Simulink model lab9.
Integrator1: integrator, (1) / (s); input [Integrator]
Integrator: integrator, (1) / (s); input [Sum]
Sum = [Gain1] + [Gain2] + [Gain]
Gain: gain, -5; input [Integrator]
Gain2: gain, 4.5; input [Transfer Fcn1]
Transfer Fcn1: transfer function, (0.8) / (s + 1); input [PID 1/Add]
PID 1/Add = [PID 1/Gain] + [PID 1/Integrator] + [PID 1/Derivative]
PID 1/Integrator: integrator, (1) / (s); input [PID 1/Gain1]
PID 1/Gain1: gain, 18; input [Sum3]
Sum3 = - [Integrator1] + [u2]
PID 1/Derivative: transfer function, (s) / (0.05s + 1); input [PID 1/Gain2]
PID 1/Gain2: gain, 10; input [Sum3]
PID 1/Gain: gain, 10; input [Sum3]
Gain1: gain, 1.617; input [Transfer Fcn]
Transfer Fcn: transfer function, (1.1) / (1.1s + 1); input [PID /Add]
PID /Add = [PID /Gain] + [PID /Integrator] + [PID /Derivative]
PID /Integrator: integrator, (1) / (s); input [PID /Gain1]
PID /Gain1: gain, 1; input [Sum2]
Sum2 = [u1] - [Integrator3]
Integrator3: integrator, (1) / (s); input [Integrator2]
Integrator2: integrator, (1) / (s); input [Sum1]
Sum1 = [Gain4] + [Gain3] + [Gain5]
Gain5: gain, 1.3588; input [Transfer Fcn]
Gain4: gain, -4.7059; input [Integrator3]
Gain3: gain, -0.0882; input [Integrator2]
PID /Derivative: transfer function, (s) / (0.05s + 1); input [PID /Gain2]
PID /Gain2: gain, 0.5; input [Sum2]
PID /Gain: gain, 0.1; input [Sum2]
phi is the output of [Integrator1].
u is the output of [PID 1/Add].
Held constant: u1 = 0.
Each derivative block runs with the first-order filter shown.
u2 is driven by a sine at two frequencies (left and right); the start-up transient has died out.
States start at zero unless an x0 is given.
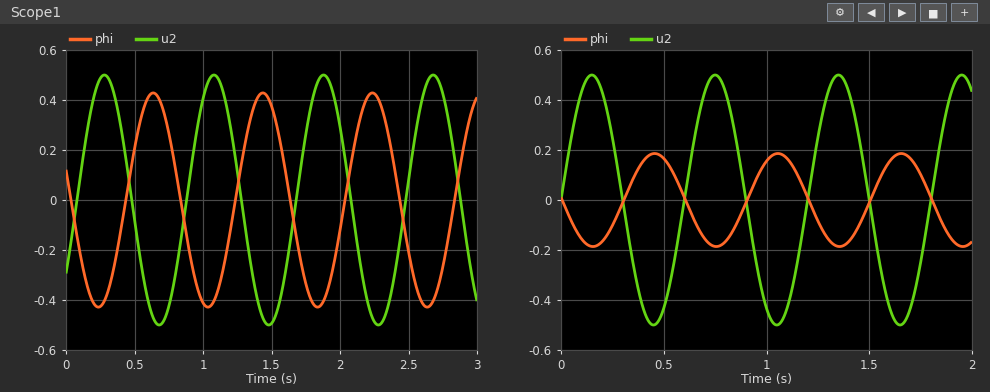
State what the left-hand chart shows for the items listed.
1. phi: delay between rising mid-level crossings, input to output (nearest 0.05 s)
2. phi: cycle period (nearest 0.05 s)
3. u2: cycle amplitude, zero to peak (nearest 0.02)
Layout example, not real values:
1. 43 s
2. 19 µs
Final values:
1. 0.35 s
2. 0.80 s
3. 0.50
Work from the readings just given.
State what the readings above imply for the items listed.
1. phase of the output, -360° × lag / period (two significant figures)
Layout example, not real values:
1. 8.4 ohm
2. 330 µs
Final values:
1. -160°
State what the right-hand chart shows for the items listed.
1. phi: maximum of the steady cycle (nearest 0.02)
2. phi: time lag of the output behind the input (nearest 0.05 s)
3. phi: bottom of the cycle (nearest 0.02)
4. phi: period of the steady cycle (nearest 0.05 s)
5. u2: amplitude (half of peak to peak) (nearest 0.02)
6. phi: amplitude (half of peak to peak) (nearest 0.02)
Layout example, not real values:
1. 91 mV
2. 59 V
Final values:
1. 0.18
2. 0.30 s
3. -0.18
4. 0.60 s
5. 0.50
6. 0.18
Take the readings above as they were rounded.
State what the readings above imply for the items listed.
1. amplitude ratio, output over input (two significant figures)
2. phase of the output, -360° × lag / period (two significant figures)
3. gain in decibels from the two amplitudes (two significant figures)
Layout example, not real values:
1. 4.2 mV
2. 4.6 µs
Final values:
1. 0.36
2. -180°
3. -8.9 dB
